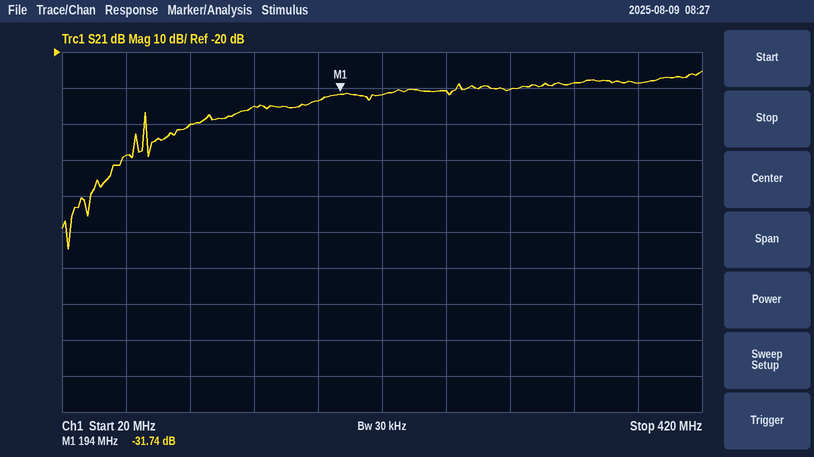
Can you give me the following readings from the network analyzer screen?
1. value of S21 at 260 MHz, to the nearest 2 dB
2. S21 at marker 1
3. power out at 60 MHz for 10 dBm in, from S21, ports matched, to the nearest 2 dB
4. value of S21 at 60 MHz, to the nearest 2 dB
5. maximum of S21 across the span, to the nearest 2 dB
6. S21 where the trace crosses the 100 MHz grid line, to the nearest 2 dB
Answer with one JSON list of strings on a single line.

["-30 dB", "-31.74 dB", "-38 dBm", "-48 dB", "-26 dB", "-40 dB"]
